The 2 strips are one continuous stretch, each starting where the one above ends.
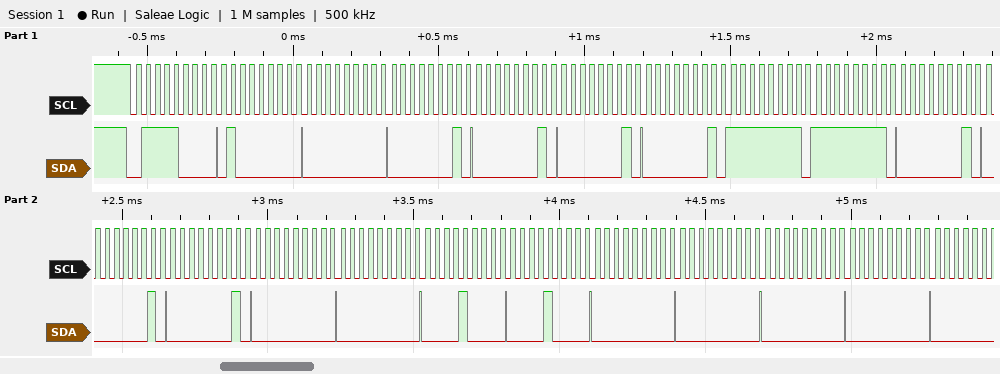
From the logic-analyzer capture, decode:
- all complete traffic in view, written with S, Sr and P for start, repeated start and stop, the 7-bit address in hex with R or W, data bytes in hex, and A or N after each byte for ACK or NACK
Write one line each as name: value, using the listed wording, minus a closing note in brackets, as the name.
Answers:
all complete traffic in view, written with S, Sr and P for start, repeated start and stop, the 7-bit address in hex with R or W, data bytes in hex, and A or N after each byte for ACK or NACK: S 3CW A 40 A 00 A 01 A 01 A 01 A 01 A FF A FF A 01 A 01 A 01 A 00 A 00 A 08 A 08 A 00 A 00 A 00 A 00 A
